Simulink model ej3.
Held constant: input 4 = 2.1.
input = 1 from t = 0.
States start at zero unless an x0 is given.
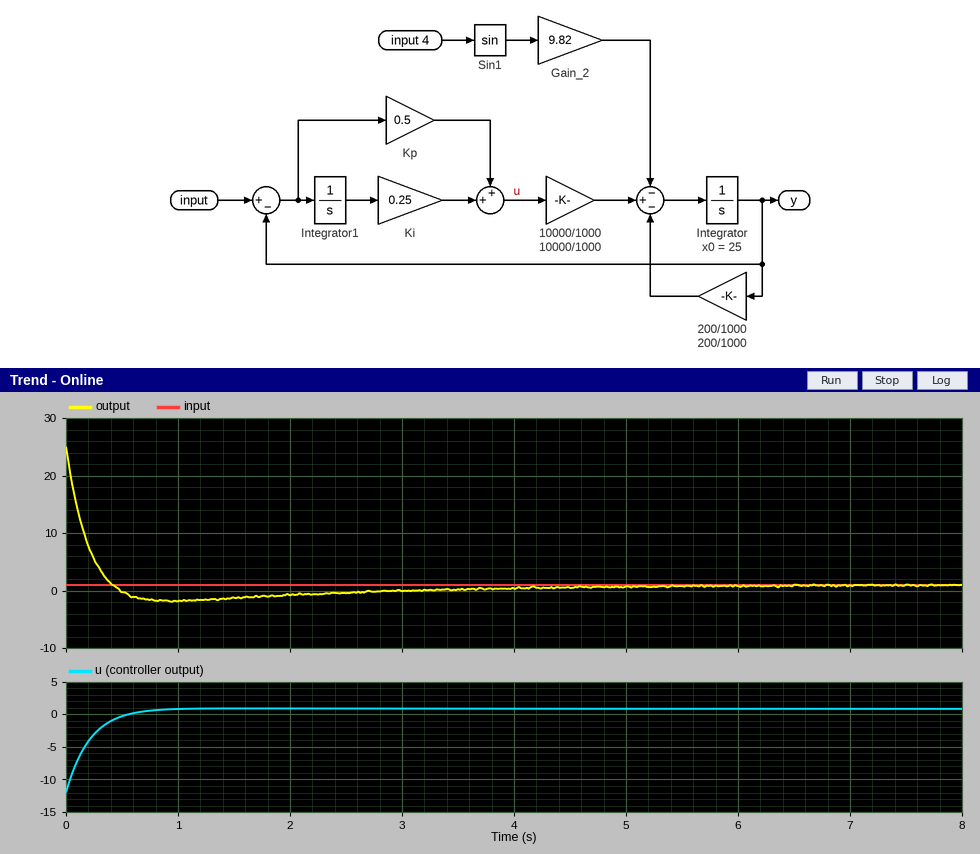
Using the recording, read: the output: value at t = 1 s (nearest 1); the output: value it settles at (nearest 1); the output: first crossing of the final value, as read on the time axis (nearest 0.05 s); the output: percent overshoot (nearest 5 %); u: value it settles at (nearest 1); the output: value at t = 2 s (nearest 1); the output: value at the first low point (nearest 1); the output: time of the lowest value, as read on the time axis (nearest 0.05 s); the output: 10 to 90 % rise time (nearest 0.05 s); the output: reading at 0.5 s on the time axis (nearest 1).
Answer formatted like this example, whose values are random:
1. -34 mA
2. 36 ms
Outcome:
1. -2
2. 1
3. 0.40 s
4. 10 %
5. 1
6. -1
7. -2
8. 0.95 s
9. 0.30 s
10. 0
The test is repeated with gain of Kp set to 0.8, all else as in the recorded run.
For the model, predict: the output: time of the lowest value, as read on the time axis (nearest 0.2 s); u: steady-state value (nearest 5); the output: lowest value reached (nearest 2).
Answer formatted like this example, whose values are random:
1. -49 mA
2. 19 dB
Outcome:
1. 0.8 s
2. 0
3. 0
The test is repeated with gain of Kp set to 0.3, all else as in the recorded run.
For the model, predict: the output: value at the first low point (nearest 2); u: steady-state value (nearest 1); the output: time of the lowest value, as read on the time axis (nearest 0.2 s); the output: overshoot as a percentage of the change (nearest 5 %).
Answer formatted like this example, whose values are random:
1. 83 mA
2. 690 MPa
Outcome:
1. -4
2. 1
3. 1.2 s
4. 20 %
